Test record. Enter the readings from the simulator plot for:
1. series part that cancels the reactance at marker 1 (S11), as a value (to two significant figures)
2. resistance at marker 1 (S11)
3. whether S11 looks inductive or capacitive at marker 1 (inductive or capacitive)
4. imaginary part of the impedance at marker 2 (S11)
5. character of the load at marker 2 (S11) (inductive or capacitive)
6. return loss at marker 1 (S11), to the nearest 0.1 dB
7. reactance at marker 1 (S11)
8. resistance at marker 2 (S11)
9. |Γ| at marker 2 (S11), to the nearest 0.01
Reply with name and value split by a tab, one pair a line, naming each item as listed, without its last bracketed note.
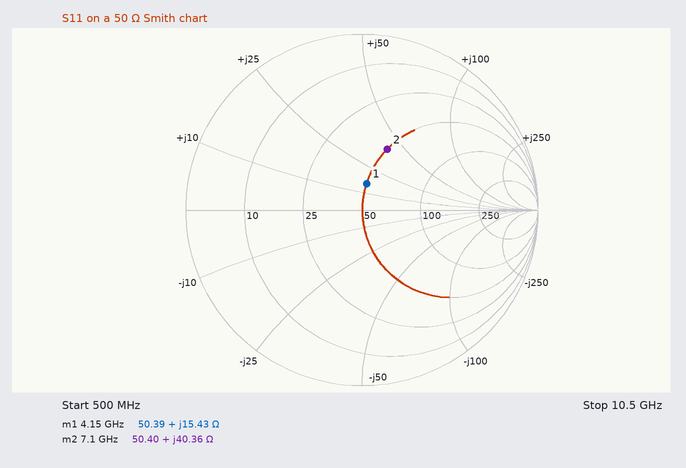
series part that cancels the reactance at marker 1 (S11), as a value	2.5 pF
resistance at marker 1	50.39 Ω
whether S11 looks inductive or capacitive at marker 1	inductive
imaginary part of the impedance at marker 2	+40.36 Ω
character of the load at marker 2 (S11)	inductive
return loss at marker 1 (S11), to the nearest 0.1 dB	16.4 dB
reactance at marker 1	+15.43 Ω
resistance at marker 2	50.40 Ω
|Γ| at marker 2 (S11), to the nearest 0.01	0.37
